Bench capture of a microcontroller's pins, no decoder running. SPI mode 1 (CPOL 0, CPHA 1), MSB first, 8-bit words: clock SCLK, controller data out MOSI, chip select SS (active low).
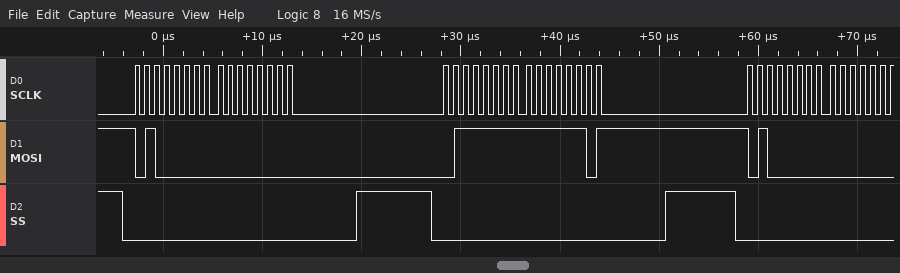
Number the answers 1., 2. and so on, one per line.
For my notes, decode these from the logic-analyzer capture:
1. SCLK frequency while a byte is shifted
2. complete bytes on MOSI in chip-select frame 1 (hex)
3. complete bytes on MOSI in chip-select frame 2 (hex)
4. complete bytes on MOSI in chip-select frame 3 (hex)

1. 1 MHz
2. 40 00
3. 7F FD
4. 40
